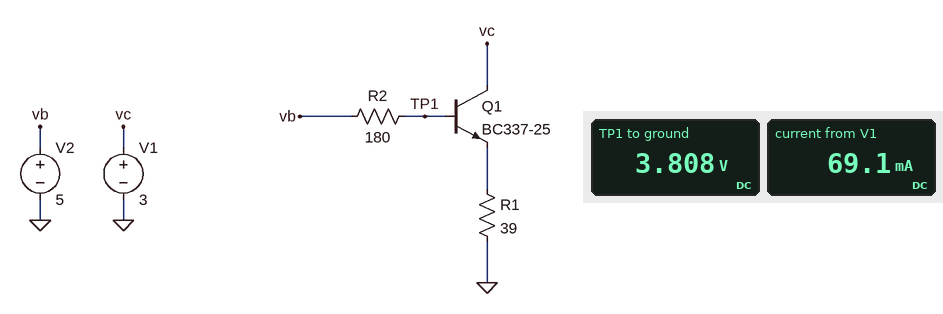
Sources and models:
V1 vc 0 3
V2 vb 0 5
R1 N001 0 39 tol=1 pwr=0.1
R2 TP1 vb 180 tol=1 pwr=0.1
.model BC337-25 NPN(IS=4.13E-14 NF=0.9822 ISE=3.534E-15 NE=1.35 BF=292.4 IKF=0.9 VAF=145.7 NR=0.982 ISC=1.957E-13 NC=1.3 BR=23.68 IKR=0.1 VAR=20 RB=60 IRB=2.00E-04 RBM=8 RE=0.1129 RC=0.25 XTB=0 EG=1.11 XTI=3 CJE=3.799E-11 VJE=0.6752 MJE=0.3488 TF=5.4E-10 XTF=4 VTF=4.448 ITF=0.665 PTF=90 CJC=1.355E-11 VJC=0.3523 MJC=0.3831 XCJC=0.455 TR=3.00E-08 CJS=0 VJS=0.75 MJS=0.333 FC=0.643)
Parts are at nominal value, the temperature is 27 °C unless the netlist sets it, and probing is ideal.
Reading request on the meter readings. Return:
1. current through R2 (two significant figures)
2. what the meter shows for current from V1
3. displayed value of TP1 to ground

6.6 mA
69.1 mA
3.808 V
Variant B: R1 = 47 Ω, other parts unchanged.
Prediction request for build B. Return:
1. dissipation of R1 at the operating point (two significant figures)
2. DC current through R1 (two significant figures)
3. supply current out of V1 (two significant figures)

190 mW
63 mA
56 mA
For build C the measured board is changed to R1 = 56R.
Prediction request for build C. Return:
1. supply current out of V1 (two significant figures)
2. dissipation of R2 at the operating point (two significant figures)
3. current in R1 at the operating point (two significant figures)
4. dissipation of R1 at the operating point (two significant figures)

46 mA
7.8 mW
53 mA
160 mW
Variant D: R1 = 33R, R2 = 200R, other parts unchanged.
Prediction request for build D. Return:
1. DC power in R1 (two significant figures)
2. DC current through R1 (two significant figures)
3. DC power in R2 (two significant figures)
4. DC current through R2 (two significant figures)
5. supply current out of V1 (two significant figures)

260 mW
89 mA
7.3 mW
6.0 mA
83 mA
